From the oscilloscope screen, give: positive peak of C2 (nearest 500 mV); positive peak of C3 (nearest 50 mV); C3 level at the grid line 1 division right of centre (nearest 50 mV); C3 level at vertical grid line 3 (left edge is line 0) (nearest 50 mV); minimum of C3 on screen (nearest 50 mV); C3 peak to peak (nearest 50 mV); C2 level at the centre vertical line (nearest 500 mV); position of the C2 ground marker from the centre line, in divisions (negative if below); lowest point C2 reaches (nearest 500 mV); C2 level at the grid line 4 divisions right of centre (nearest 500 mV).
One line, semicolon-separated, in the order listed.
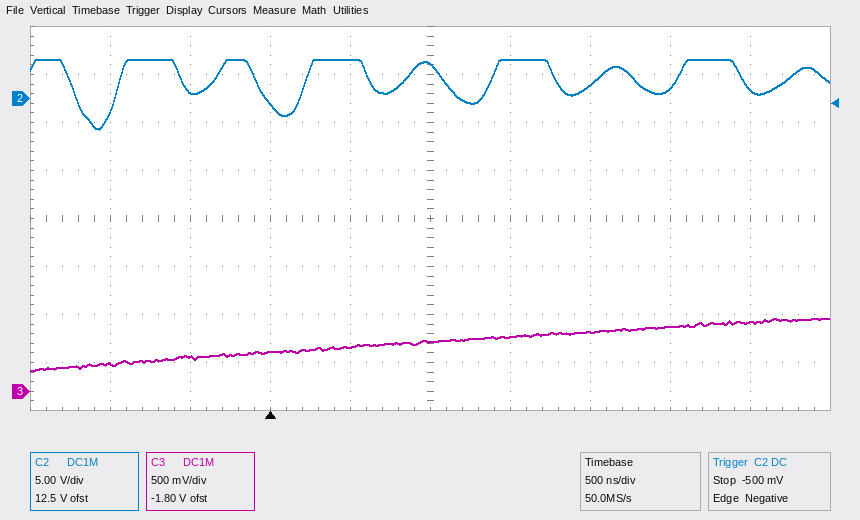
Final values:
4.0 V; 750 mV; 550 mV; 400 mV; 200 mV; 550 mV; 3.5 V; +2.5 div; -3.0 V; 1.0 V
